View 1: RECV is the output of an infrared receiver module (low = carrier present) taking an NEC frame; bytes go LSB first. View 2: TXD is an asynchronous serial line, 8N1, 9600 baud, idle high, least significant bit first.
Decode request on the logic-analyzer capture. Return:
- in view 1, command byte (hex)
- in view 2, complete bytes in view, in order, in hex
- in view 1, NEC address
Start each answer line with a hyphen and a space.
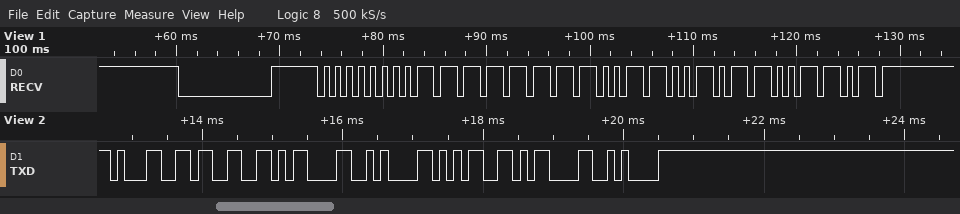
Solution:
- 0x4C
- 31 33 0D 0A 35 0D 0A
- 0x00
